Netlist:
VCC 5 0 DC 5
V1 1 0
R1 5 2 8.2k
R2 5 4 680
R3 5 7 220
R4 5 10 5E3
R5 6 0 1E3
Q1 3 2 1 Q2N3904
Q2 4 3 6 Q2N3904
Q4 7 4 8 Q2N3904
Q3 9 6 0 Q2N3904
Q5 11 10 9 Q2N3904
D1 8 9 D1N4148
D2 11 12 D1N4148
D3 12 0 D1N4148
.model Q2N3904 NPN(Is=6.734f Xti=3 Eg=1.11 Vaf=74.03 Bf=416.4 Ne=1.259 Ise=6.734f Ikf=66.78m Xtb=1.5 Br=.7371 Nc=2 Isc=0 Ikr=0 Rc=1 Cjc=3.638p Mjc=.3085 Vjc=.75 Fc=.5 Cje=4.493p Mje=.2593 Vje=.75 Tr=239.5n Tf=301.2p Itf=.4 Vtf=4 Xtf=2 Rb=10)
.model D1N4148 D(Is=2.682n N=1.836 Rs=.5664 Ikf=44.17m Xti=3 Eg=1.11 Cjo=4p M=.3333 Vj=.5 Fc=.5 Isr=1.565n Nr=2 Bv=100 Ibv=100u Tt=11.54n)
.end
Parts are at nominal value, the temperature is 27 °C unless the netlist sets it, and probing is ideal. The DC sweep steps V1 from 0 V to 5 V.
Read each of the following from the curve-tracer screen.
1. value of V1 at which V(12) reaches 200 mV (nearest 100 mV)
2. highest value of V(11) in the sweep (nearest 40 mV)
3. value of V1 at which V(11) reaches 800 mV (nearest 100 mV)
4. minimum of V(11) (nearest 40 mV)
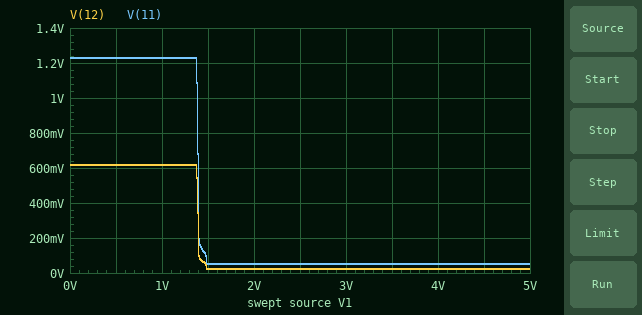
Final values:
1.4 V
1.24 V
1.4 V
40 mV
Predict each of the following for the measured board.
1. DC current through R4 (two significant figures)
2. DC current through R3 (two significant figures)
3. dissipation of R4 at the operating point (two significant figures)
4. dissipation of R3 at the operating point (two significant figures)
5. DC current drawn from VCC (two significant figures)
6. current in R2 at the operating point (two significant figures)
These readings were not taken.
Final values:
620 µA
450 µA
1.9 mW
45 µW
1.6 mA
3.8 µA
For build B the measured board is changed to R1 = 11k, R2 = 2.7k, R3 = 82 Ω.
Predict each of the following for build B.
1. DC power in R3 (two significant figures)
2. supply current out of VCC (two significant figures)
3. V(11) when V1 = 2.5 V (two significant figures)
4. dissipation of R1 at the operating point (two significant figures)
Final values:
17 µW
1.5 mA
55 mV
1.7 mW
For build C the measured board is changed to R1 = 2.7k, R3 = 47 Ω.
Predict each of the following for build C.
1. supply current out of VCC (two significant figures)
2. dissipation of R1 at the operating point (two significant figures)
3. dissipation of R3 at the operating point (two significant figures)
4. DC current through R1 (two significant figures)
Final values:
2.7 mA
6.8 mW
9.6 µW
1.6 mA
